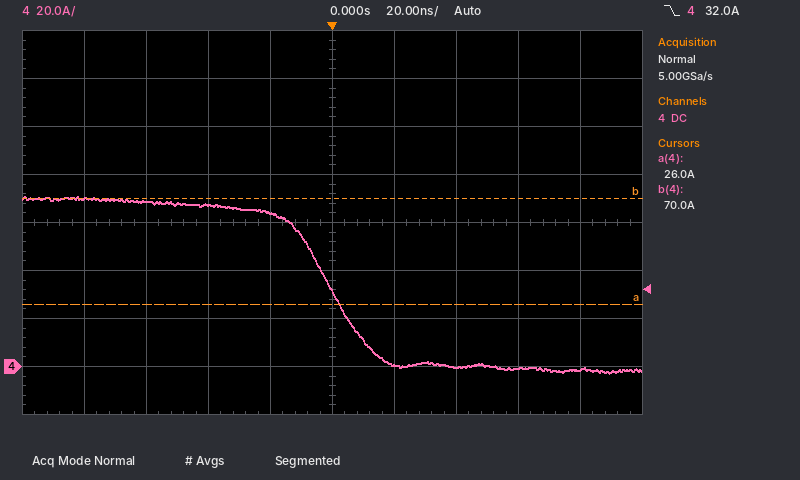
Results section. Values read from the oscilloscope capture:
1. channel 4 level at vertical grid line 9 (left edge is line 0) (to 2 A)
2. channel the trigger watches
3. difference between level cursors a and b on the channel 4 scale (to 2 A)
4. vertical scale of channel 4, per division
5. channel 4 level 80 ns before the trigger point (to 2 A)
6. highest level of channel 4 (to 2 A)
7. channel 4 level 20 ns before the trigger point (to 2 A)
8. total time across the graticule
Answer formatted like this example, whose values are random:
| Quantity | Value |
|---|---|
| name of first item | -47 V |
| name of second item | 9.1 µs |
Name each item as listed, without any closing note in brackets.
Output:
| Quantity | Value |
|---|---|
| channel 4 level at vertical grid line 9 (left edge is line 0) | -2 A |
| channel the trigger watches | channel 4 |
| difference between level cursors a and b on the channel 4 scale | 44 A |
| vertical scale of channel 4, per division | 20 A |
| channel 4 level 80 ns before the trigger point | 70 A |
| highest level of channel 4 | 70 A |
| channel 4 level 20 ns before the trigger point | 64 A |
| total time across the graticule | 200 ns |
